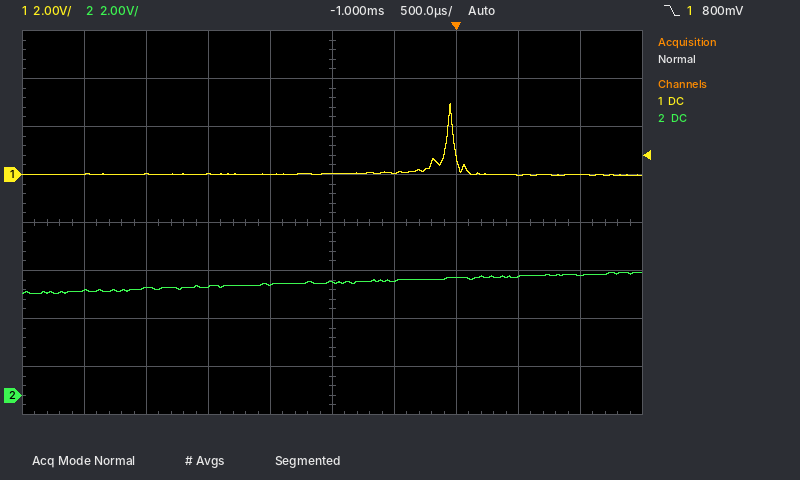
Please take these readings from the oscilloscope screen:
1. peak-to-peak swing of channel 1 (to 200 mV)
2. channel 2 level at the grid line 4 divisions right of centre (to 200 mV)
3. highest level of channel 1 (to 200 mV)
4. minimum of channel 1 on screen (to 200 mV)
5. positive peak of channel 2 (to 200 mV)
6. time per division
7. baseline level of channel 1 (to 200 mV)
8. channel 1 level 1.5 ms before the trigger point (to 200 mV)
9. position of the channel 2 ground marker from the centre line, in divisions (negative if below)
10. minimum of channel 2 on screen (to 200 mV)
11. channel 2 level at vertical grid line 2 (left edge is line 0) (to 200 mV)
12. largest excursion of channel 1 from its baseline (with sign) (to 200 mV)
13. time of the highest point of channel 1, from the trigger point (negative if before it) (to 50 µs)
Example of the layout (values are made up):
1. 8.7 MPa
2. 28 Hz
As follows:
1. 3.0 V
2. 5.0 V
3. 3.0 V
4. 0.0 V
5. 5.2 V
6. 500 µs
7. 0.0 V
8. 0.0 V
9. -3.6 div
10. 4.2 V
11. 4.4 V
12. +3.0 V
13. -50 µs
